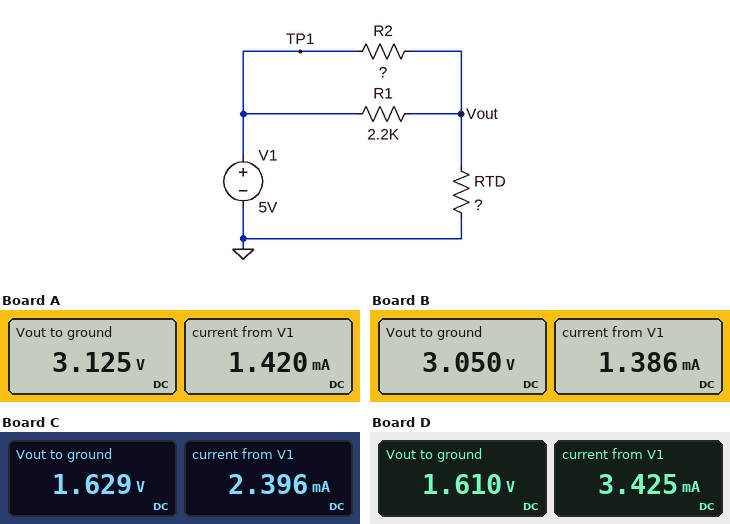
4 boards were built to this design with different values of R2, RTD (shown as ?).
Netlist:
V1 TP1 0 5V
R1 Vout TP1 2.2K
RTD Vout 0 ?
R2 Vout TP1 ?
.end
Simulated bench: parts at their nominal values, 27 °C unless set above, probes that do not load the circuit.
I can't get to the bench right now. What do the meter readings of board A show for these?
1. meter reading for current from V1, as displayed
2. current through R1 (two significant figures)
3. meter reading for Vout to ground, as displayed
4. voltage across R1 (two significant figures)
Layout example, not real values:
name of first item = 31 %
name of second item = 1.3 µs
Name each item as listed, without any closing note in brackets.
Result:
meter reading for current from V1, as displayed = 1.420 mA
current through R1 = 850 µA
meter reading for Vout to ground, as displayed = 3.125 V
voltage across R1 = 1.9 V
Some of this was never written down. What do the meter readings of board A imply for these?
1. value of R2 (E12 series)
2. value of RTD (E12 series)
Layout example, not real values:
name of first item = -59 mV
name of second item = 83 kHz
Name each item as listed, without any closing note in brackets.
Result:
value of R2 = 3.3 kΩ
value of RTD = 2.2 kΩ
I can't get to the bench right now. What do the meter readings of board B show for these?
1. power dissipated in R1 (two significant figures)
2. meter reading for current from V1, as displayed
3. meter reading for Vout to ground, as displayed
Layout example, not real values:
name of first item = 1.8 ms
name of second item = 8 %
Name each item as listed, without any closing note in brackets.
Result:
power dissipated in R1 = 1.7 mW
meter reading for current from V1, as displayed = 1.386 mA
meter reading for Vout to ground, as displayed = 3.050 V
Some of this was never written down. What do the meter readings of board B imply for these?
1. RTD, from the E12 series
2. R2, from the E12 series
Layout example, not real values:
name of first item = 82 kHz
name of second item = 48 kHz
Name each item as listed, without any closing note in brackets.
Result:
RTD, from the E12 series = 2.2 kΩ
R2, from the E12 series = 3.9 kΩ
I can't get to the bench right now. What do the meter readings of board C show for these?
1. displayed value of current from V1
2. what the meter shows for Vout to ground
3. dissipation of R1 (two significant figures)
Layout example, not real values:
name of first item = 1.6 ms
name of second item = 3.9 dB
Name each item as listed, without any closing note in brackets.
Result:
displayed value of current from V1 = 2.396 mA
what the meter shows for Vout to ground = 1.629 V
dissipation of R1 = 5.2 mW
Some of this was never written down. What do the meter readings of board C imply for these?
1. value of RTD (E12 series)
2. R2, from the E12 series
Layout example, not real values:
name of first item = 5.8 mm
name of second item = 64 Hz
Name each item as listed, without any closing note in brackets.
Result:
value of RTD = 680 Ω
R2, from the E12 series = 3.9 kΩ
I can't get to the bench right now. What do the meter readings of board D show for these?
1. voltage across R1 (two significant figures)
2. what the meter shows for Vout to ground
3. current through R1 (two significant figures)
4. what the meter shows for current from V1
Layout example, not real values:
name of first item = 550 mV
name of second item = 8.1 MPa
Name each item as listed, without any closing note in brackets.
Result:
voltage across R1 = 3.4 V
what the meter shows for Vout to ground = 1.610 V
current through R1 = 1.5 mA
what the meter shows for current from V1 = 3.425 mA
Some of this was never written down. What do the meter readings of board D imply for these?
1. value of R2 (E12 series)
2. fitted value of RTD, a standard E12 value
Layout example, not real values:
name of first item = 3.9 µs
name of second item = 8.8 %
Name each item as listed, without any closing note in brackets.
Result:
value of R2 = 1.8 kΩ
fitted value of RTD, a standard E12 value = 470 Ω
